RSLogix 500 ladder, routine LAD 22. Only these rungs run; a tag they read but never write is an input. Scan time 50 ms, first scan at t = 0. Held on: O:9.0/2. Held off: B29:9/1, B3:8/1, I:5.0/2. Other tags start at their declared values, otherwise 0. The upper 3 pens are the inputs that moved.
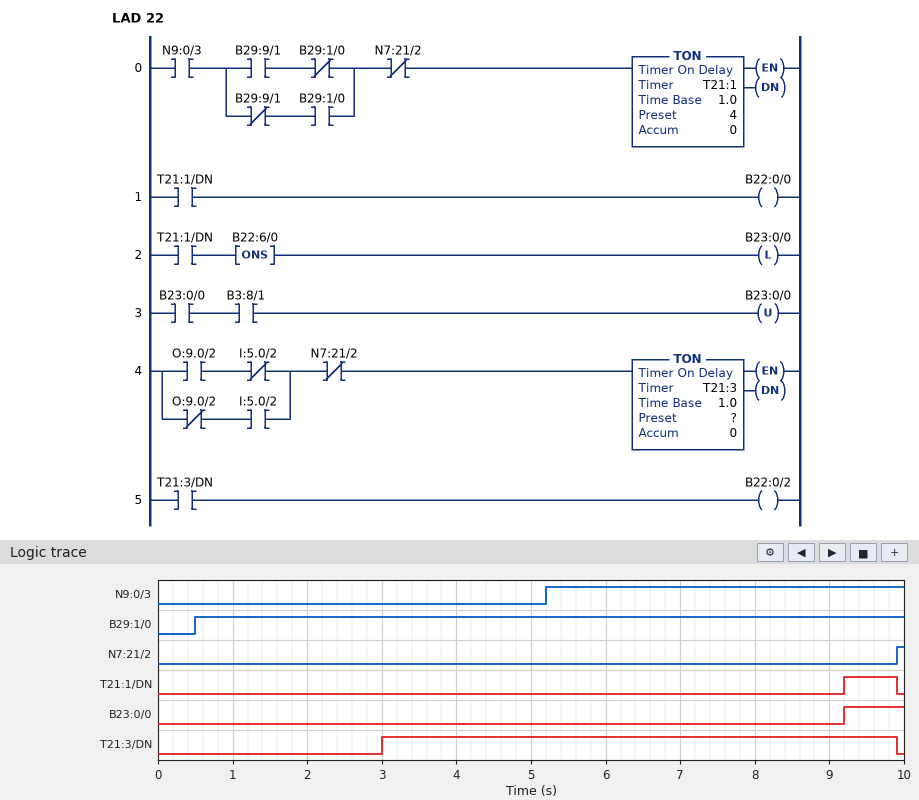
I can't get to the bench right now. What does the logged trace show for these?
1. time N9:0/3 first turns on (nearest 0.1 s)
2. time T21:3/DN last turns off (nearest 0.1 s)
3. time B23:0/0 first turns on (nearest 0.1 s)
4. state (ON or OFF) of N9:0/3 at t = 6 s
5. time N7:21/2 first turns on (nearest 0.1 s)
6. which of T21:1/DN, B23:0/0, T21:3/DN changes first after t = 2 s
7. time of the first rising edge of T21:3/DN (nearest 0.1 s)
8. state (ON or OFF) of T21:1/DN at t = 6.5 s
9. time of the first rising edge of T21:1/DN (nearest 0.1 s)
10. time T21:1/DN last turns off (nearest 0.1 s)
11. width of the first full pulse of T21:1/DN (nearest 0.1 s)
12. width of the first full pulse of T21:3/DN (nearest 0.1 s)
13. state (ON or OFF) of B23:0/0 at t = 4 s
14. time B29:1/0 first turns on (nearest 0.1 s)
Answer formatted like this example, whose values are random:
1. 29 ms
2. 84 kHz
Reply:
1. 5.2 s
2. 9.9 s
3. 9.2 s
4. ON
5. 9.9 s
6. T21:3/DN
7. 3.0 s
8. OFF
9. 9.2 s
10. 9.9 s
11. 0.7 s
12. 6.9 s
13. OFF
14. 0.5 s
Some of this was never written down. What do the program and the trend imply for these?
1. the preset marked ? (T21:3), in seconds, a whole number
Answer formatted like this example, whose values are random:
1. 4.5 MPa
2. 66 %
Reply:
1. 3 s
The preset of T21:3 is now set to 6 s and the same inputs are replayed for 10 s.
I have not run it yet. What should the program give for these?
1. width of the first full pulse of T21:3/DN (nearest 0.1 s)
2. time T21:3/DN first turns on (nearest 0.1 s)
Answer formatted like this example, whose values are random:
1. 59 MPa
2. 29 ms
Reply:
1. 3.9 s
2. 6.0 s
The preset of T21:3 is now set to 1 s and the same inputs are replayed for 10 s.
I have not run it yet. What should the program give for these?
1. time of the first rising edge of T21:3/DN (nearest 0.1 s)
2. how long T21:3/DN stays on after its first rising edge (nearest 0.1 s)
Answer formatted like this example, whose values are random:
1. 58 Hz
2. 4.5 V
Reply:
1. 1.0 s
2. 8.9 s
